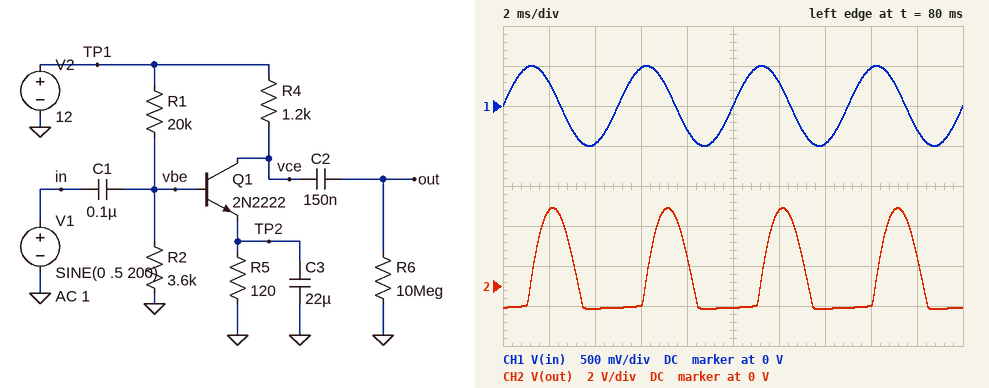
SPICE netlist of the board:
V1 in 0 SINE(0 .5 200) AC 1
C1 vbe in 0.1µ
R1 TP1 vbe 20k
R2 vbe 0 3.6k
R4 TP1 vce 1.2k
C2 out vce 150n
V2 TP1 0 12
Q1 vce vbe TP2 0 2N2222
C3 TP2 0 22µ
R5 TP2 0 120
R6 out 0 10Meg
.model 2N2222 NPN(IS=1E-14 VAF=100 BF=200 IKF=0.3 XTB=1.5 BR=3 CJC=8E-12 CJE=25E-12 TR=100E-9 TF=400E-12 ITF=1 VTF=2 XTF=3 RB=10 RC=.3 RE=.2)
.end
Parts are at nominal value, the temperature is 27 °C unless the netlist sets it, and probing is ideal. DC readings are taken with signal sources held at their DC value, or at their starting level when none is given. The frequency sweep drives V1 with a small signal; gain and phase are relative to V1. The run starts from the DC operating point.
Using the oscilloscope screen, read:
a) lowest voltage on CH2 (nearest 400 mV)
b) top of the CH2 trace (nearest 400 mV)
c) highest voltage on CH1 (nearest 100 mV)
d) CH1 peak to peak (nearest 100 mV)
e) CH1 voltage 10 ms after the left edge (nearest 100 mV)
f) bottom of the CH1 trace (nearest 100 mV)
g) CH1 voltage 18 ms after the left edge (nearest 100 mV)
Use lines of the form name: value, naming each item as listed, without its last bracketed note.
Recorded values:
lowest voltage on CH2: -1.2 V
top of the CH2 trace: 4.0 V
highest voltage on CH1: 500 mV
CH1 peak to peak: 1.0 V
CH1 voltage 10 ms after the left edge: 0 V
bottom of the CH1 trace: -500 mV
CH1 voltage 18 ms after the left edge: -300 mV
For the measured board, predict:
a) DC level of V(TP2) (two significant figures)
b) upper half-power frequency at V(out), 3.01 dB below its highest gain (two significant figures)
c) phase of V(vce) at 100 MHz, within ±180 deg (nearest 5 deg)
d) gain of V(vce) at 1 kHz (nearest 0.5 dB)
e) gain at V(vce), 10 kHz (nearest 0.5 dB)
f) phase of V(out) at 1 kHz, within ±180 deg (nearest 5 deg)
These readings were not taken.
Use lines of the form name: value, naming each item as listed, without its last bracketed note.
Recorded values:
DC level of V(TP2): 990 mV
upper half-power frequency at V(out), 3.01 dB below its highest gain: 5.4 MHz
phase of V(vce) at 100 MHz, within ±180 deg: 80 deg
gain of V(vce) at 1 kHz: 36.0 dB
gain at V(vce), 10 kHz: 49.0 dB
phase of V(out) at 1 kHz, within ±180 deg: -90 deg
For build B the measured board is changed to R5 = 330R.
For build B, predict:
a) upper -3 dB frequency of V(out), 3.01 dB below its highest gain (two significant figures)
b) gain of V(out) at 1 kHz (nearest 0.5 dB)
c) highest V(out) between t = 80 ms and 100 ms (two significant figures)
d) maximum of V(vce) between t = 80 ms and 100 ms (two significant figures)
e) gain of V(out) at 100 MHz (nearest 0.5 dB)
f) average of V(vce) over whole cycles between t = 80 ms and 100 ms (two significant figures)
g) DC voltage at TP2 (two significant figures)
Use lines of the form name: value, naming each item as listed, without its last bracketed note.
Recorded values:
upper -3 dB frequency of V(out), 3.01 dB below its highest gain: 15 MHz
gain of V(out) at 1 kHz: 35.5 dB
highest V(out) between t = 80 ms and 100 ms: 3.7 V
maximum of V(vce) between t = 80 ms and 100 ms: 12 V
gain of V(out) at 100 MHz: 26.5 dB
average of V(vce) over whole cycles between t = 80 ms and 100 ms: 8.0 V
DC voltage at TP2: 1.1 V
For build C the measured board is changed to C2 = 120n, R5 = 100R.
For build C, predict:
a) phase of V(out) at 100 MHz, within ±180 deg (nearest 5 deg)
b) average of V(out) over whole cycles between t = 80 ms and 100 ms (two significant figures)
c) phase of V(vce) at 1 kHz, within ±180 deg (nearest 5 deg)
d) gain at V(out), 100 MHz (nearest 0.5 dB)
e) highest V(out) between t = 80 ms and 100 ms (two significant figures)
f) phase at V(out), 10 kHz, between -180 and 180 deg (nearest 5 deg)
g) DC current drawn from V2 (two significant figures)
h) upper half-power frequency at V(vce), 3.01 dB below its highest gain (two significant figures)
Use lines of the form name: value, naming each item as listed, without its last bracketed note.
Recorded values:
phase of V(out) at 100 MHz, within ±180 deg: 55 deg
average of V(out) over whole cycles between t = 80 ms and 100 ms: 530 mV
phase of V(vce) at 1 kHz, within ±180 deg: -90 deg
gain at V(out), 100 MHz: -4.5 dB
highest V(out) between t = 80 ms and 100 ms: 2.8 V
phase at V(out), 10 kHz, between -180 and 180 deg: -100 deg
DC current drawn from V2: 9.6 mA
upper half-power frequency at V(vce), 3.01 dB below its highest gain: 1.2 MHz
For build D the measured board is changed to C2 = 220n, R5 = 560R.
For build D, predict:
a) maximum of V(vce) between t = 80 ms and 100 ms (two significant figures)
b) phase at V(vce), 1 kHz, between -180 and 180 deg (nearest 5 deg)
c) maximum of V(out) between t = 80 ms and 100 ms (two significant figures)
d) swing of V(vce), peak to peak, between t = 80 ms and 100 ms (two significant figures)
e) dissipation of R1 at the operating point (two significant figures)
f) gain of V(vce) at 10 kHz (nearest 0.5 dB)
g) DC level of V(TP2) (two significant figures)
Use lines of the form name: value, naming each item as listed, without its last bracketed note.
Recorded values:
maximum of V(vce) between t = 80 ms and 100 ms: 12 V
phase at V(vce), 1 kHz, between -180 and 180 deg: -115 deg
maximum of V(out) between t = 80 ms and 100 ms: 2.4 V
swing of V(vce), peak to peak, between t = 80 ms and 100 ms: 6.6 V
dissipation of R1 at the operating point: 5.2 mW
gain of V(vce) at 10 kHz: 39.0 dB
DC level of V(TP2): 1.1 V
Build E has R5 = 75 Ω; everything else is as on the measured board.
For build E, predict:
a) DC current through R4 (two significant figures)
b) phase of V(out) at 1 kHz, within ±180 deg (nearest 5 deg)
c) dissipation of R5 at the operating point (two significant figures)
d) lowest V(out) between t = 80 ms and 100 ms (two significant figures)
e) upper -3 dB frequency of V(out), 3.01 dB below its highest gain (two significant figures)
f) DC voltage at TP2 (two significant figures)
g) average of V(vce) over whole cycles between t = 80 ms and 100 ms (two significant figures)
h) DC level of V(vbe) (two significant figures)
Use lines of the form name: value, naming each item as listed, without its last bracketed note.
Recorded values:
DC current through R4: 9.3 mA
phase of V(out) at 1 kHz, within ±180 deg: -90 deg
dissipation of R5 at the operating point: 6.7 mW
lowest V(out) between t = 80 ms and 100 ms: -13 mV
upper -3 dB frequency of V(out), 3.01 dB below its highest gain: 1.1 MHz
DC voltage at TP2: 710 mV
average of V(vce) over whole cycles between t = 80 ms and 100 ms: 810 mV
DC level of V(vbe): 1.4 V
